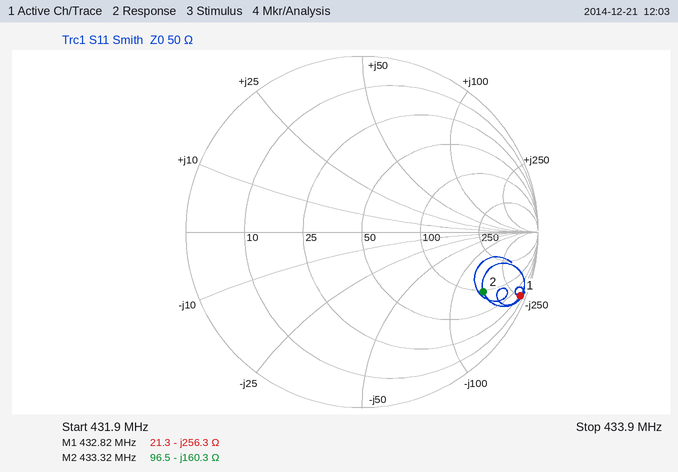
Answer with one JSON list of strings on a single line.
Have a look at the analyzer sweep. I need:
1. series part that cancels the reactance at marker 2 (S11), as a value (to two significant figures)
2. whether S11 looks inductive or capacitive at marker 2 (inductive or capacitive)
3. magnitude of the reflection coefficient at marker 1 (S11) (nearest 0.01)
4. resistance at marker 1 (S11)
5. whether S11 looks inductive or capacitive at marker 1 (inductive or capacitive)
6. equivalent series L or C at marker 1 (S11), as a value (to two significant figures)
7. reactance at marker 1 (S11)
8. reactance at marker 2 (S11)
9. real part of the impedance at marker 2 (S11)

["59 nH", "capacitive", "0.97", "21.3 Ω", "capacitive", "1.4 pF", "-256.3 Ω", "-160.3 Ω", "96.5 Ω"]
